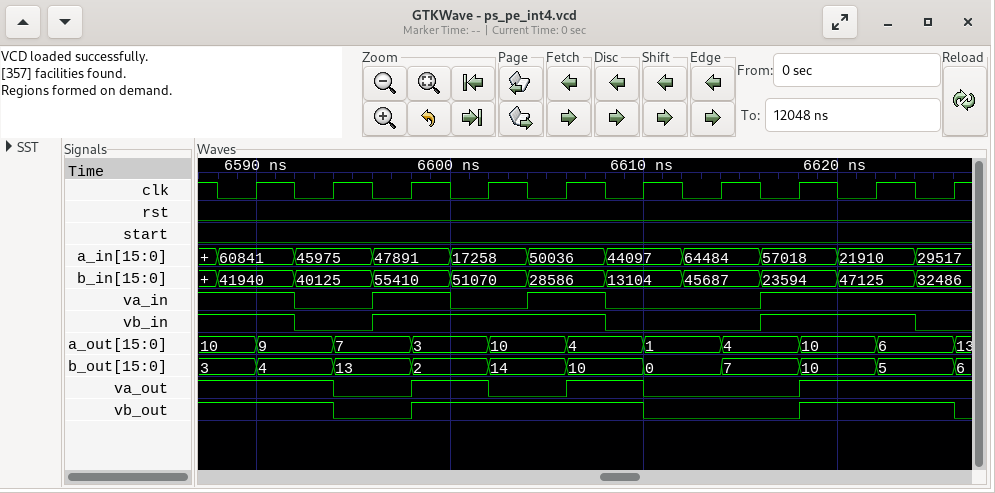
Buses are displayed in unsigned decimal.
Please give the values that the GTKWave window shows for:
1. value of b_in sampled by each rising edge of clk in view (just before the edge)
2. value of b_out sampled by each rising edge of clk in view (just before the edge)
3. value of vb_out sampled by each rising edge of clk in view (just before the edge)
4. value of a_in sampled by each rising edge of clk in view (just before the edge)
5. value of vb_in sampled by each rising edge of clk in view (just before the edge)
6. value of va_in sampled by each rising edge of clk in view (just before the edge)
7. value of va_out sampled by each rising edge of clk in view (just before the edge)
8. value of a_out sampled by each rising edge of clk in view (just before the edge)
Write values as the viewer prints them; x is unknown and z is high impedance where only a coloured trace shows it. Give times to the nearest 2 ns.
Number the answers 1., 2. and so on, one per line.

1. 41940, 40125, 55410, 51070, 28586, 13104, 45687, 23594, 47125, 32486
2. 3, 4, 13, 2, 14, 10, 0, 7, 10, 5
3. 1 1 0 1 1 1 0 0 1 1
4. 60841, 45975, 47891, 17258, 50036, 44097, 64484, 57018, 21910, 29517
5. 1 0 1 1 1 0 0 1 1 0
6. 1 0 1 0 1 0 0 1 1 1
7. 1 1 0 1 0 1 0 0 1 1
8. 10, 9, 7, 3, 10, 4, 1, 4, 10, 6
